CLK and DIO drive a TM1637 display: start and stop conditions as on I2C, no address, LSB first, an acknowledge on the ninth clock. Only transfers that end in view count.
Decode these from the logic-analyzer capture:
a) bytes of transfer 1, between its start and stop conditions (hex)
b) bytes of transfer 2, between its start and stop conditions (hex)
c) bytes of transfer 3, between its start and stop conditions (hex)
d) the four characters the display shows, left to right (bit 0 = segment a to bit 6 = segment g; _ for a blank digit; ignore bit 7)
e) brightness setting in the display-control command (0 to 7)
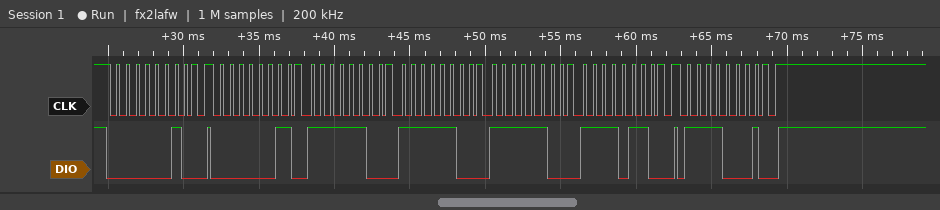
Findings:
40
C0 3F 3F 3F 6F
8F
0009
7
